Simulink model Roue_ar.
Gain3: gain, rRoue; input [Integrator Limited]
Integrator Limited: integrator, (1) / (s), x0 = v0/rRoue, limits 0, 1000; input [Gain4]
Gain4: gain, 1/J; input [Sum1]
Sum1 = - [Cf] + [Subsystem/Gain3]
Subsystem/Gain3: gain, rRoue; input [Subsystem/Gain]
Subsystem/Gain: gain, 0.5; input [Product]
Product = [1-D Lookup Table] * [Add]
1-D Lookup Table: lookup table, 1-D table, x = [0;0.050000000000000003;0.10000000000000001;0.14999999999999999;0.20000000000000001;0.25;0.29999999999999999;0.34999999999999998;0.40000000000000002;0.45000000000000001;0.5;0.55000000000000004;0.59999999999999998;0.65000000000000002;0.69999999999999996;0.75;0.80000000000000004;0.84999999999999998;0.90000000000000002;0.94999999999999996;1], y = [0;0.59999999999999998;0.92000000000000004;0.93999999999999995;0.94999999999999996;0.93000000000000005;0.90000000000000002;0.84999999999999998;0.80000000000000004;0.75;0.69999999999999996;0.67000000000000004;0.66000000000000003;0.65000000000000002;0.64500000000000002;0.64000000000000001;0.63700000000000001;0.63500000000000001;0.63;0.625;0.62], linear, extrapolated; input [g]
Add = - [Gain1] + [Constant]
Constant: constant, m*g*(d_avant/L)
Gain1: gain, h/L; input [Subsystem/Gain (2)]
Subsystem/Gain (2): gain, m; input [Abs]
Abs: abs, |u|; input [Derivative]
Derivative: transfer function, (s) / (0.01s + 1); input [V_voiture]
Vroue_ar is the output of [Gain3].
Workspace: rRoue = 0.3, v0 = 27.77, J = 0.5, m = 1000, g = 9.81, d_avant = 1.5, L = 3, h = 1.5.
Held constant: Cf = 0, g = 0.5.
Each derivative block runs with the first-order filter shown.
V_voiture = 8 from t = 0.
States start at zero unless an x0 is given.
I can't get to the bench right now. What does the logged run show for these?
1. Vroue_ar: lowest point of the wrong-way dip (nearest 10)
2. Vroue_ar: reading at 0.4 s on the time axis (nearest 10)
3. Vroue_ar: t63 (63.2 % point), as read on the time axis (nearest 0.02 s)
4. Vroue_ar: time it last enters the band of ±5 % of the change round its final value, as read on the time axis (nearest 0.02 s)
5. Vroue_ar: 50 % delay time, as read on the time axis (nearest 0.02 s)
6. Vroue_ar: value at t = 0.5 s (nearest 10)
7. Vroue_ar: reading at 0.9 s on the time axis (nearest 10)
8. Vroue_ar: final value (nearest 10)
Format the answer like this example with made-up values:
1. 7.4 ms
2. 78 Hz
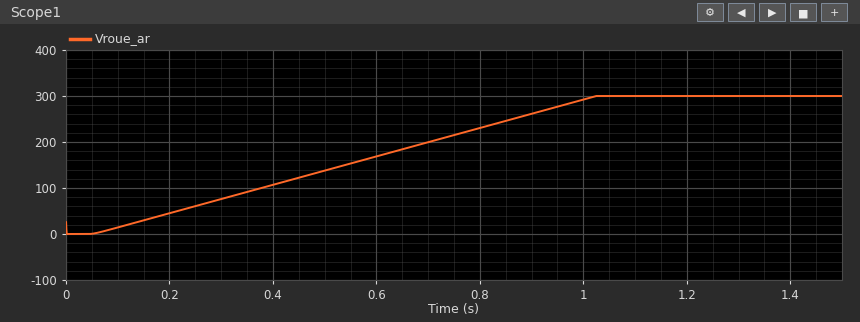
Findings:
1. 0
2. 110
3. 0.70 s
4. 0.98 s
5. 0.58 s
6. 140
7. 260
8. 300
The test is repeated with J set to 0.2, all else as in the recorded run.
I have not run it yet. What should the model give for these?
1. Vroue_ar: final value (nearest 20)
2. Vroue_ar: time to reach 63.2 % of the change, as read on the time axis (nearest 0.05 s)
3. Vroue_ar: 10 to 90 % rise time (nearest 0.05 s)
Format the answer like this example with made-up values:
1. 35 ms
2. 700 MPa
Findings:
1. 300
2. 0.30 s
3. 0.30 s
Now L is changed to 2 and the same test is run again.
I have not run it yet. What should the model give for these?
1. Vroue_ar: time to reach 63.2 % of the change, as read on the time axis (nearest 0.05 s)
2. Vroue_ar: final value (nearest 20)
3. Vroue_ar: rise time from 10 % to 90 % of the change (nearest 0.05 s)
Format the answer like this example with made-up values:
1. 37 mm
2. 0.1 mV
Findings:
1. 0.50 s
2. 300
3. 0.45 s
